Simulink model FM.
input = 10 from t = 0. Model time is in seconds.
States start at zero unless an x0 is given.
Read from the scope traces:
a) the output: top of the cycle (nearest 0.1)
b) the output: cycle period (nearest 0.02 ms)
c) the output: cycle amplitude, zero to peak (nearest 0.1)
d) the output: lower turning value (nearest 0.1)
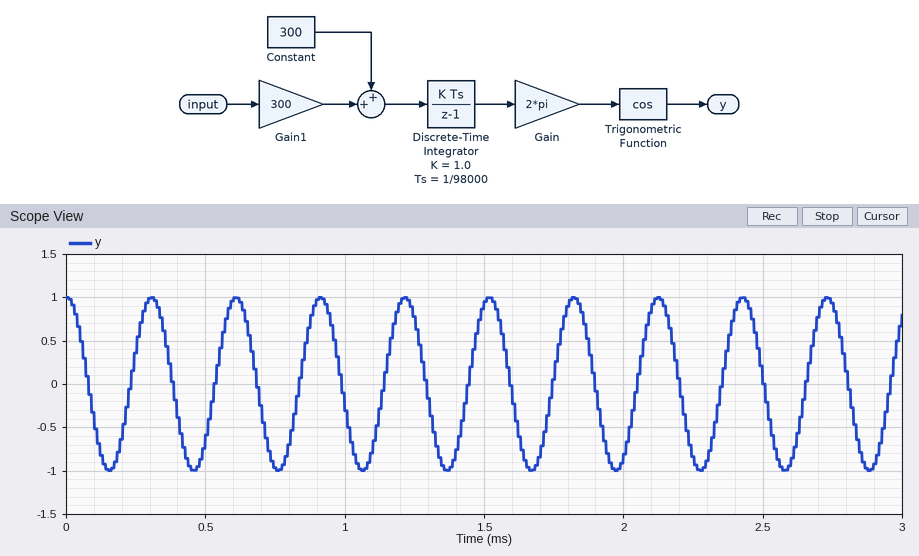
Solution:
1.0
0.30 ms
1.0
-1.0
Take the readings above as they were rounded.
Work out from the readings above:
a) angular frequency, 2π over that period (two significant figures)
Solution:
21 rad/ms
